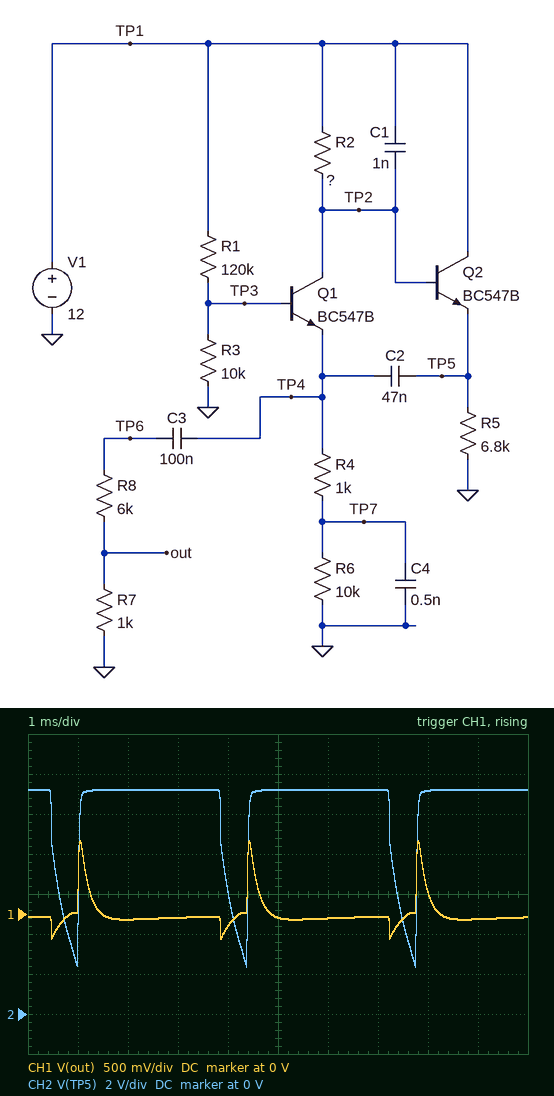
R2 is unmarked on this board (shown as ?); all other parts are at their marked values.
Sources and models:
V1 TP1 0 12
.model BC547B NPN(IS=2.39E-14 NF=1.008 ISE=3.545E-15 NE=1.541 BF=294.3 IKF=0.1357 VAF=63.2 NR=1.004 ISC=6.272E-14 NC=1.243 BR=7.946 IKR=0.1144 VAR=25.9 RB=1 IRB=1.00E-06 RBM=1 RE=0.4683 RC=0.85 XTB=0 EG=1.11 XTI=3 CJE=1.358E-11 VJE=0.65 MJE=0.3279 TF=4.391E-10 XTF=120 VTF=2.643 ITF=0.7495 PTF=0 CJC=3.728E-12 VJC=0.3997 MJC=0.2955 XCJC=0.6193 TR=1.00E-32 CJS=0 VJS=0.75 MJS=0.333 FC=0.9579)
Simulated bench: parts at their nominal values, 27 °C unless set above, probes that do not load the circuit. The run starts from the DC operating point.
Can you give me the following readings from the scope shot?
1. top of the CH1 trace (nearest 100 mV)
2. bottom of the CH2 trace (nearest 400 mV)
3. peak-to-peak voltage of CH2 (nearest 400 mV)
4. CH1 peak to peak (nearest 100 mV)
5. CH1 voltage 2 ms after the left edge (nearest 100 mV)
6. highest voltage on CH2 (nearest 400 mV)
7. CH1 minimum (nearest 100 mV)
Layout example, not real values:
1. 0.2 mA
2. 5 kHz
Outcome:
1. 900 mV
2. 2.4 V
3. 8.8 V
4. 1.2 V
5. -100 mV
6. 11.2 V
7. -300 mV
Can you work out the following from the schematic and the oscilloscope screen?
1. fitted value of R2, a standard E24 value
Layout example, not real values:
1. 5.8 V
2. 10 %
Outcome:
1. 22 kΩ
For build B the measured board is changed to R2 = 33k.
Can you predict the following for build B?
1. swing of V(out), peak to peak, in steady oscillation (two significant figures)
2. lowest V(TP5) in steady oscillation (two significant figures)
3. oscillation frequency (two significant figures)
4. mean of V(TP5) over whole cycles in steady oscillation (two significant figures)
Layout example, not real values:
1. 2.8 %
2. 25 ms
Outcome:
1. 1.3 V
2. 1.5 V
3. 270 Hz
4. 9.6 V
